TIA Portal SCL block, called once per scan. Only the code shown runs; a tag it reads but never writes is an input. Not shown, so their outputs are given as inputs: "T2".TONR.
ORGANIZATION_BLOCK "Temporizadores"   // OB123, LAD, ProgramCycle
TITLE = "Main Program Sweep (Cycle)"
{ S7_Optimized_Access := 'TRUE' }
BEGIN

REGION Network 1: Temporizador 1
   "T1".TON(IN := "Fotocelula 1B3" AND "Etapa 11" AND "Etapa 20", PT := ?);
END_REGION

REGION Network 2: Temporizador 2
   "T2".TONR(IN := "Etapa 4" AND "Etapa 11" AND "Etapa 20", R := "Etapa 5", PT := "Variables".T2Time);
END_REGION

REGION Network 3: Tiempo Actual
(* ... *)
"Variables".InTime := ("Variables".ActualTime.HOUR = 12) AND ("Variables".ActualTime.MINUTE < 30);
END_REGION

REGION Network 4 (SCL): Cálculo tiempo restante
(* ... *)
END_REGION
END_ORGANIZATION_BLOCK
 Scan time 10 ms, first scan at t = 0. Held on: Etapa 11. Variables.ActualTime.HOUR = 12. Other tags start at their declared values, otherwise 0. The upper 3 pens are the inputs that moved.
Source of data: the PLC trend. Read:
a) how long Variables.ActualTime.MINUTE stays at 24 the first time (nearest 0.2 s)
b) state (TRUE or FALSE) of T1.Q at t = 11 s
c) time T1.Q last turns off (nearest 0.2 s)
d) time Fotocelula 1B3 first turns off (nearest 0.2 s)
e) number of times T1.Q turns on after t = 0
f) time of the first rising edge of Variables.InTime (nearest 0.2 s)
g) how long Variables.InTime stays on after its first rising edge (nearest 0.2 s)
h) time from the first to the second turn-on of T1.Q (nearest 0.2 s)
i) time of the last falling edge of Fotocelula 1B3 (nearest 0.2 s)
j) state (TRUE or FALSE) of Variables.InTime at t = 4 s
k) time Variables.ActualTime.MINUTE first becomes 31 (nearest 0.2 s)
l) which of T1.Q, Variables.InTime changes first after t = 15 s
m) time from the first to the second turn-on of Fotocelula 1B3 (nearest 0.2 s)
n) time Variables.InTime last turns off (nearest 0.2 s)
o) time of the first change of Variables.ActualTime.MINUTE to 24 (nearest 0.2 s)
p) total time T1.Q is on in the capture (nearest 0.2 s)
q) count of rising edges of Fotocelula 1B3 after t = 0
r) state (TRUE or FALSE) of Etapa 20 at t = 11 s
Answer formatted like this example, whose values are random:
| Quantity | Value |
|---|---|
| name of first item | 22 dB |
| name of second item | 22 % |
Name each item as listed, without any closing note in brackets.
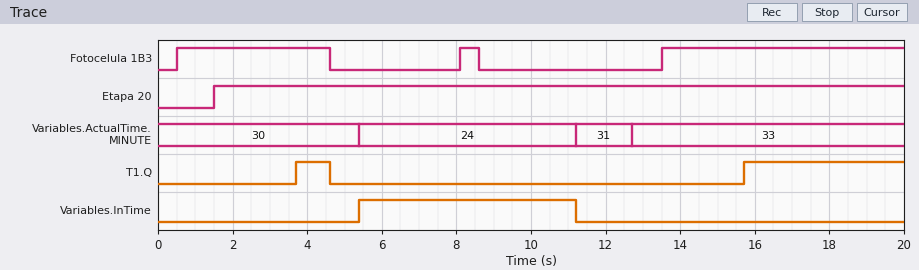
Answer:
| Quantity | Value |
|---|---|
| how long Variables.ActualTime.MINUTE stays at 24 the first time | 5.8 s |
| state (TRUE or FALSE) of T1.Q at t = 11 s | FALSE |
| time T1.Q last turns off | 4.6 s |
| time Fotocelula 1B3 first turns off | 4.6 s |
| number of times T1.Q turns on after t = 0 | 2 |
| time of the first rising edge of Variables.InTime | 5.4 s |
| how long Variables.InTime stays on after its first rising edge | 5.8 s |
| time from the first to the second turn-on of T1.Q | 12.0 s |
| time of the last falling edge of Fotocelula 1B3 | 8.6 s |
| state (TRUE or FALSE) of Variables.InTime at t = 4 s | FALSE |
| time Variables.ActualTime.MINUTE first becomes 31 | 11.2 s |
| which of T1.Q, Variables.InTime changes first after t = 15 s | T1.Q |
| time from the first to the second turn-on of Fotocelula 1B3 | 7.6 s |
| time Variables.InTime last turns off | 11.2 s |
| time of the first change of Variables.ActualTime.MINUTE to 24 | 5.4 s |
| total time T1.Q is on in the capture | 5.2 s |
| count of rising edges of Fotocelula 1B3 after t = 0 | 3 |
| state (TRUE or FALSE) of Etapa 20 at t = 11 s | TRUE |
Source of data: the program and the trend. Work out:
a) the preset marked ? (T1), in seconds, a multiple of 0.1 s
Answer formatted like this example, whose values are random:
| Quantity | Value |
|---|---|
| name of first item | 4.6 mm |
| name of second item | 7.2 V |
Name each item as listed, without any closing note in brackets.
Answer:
| Quantity | Value |
|---|---|
| the preset marked ? (T1), in seconds, a multiple of 0.1 s | 2.2 s |
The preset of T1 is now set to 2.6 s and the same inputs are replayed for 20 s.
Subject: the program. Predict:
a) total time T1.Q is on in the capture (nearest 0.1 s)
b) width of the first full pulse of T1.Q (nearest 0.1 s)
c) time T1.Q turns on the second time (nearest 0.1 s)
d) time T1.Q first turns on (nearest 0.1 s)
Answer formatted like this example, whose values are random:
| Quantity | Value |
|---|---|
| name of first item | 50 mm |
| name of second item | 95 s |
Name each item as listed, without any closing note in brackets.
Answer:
| Quantity | Value |
|---|---|
| total time T1.Q is on in the capture | 4.4 s |
| width of the first full pulse of T1.Q | 0.5 s |
| time T1.Q turns on the second time | 16.1 s |
| time T1.Q first turns on | 4.1 s |
